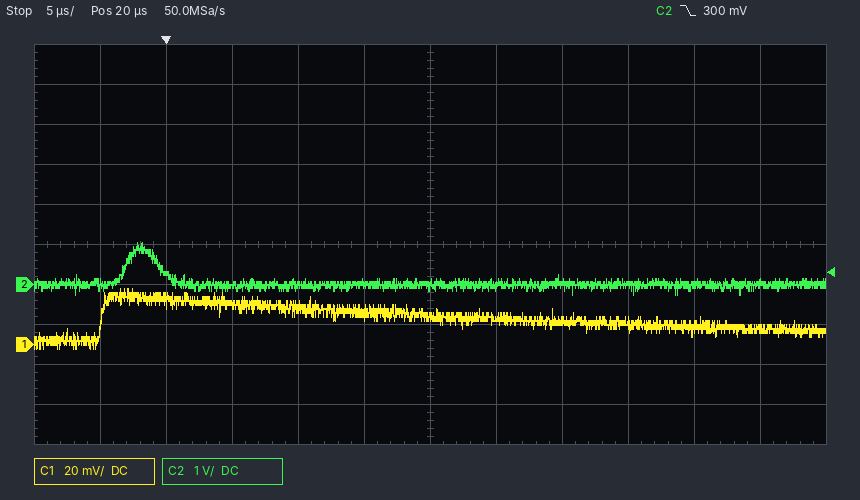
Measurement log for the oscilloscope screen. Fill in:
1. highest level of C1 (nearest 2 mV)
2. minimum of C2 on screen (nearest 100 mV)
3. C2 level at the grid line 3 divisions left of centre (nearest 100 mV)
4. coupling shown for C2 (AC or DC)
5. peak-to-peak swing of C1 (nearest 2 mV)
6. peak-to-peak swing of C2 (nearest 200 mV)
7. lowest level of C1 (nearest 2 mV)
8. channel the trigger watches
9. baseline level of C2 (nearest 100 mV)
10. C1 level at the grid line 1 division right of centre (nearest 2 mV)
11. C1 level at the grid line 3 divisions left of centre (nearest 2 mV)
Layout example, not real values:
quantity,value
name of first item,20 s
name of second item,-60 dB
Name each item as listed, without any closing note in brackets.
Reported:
quantity,value
highest level of C1,28 mV
minimum of C2 on screen,-200 mV
C2 level at the grid line 3 divisions left of centre,0.0 V
coupling shown for C2,DC
peak-to-peak swing of C1,30 mV
peak-to-peak swing of C2,1.2 V
lowest level of C1,-2 mV
channel the trigger watches,C2
baseline level of C2,0.0 V
C1 level at the grid line 1 division right of centre,14 mV
C1 level at the grid line 3 divisions left of centre,20 mV
